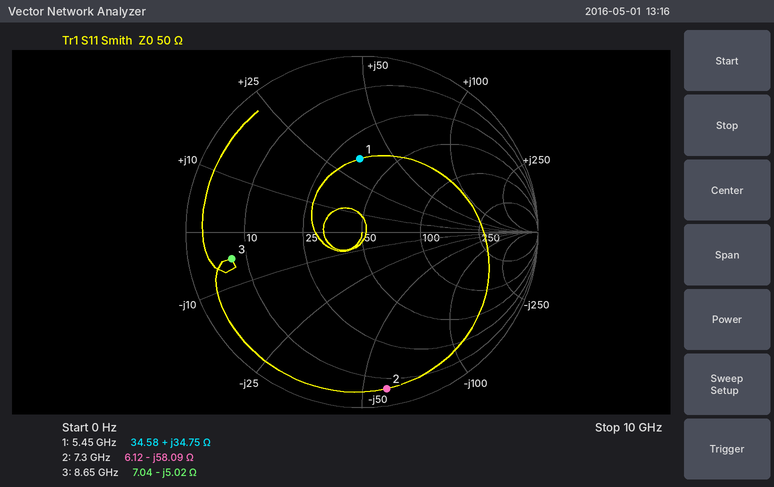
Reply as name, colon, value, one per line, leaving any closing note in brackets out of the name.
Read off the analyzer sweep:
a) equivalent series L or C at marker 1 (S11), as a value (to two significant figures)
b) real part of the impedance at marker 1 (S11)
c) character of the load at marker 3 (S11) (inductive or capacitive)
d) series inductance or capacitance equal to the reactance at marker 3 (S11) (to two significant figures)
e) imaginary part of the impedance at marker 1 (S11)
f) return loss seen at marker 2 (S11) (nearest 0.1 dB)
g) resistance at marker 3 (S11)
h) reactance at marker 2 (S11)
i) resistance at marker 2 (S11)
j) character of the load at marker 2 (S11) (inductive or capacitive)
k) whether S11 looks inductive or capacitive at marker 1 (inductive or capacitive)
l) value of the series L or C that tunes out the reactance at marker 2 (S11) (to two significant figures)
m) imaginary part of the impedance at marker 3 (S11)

equivalent series L or C at marker 1 (S11), as a value: 1.0 nH
real part of the impedance at marker 1: 34.58 Ω
character of the load at marker 3 (S11): capacitive
series inductance or capacitance equal to the reactance at marker 3 (S11): 3.7 pF
imaginary part of the impedance at marker 1: +34.75 Ω
return loss seen at marker 2 (S11): 0.9 dB
resistance at marker 3: 7.04 Ω
reactance at marker 2: -58.09 Ω
resistance at marker 2: 6.12 Ω
character of the load at marker 2 (S11): capacitive
whether S11 looks inductive or capacitive at marker 1: inductive
value of the series L or C that tunes out the reactance at marker 2 (S11): 1.3 nH
imaginary part of the impedance at marker 3: -5.02 Ω
